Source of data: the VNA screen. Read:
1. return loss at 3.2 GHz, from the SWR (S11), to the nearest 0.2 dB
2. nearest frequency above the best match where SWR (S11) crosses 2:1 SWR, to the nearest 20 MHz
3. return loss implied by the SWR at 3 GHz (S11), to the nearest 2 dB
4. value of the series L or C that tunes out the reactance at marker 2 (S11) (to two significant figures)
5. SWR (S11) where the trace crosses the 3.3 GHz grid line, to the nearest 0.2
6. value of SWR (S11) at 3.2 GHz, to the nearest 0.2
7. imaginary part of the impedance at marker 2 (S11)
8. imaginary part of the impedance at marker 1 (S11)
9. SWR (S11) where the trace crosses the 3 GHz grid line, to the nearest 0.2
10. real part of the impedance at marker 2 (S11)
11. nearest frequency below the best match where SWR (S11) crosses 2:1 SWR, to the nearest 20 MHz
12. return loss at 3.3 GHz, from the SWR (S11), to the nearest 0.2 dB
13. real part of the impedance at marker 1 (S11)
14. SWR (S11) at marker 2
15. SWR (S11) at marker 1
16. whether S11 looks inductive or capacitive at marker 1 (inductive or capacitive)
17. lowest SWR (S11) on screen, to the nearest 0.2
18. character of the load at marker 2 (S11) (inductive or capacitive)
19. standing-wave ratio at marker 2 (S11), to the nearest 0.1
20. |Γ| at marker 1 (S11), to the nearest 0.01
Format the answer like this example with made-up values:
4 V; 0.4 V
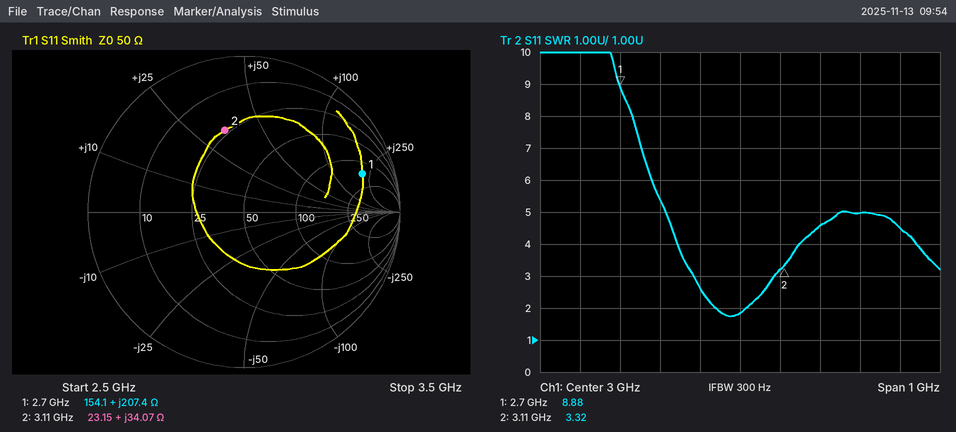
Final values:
3.8 dB; 3.02 GHz; 10 dB; 1.5 pF; 5.0; 4.6; +34.07 Ω; +207.4 Ω; 1.8; 23.15 Ω; 2.94 GHz; 3.6 dB; 154.1 Ω; 3.32; 8.88; inductive; 1.8; inductive; 3.3; 0.80
